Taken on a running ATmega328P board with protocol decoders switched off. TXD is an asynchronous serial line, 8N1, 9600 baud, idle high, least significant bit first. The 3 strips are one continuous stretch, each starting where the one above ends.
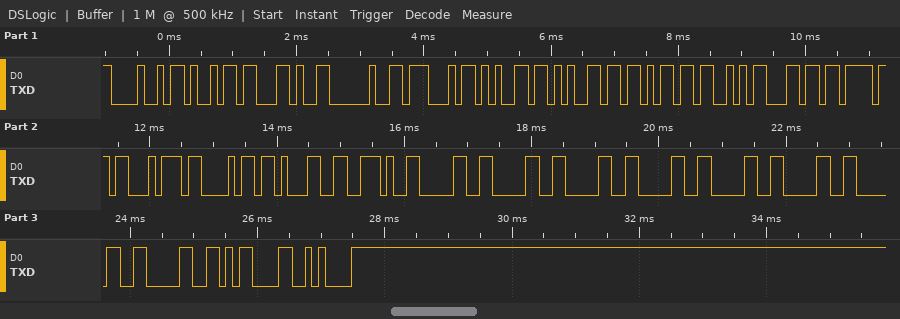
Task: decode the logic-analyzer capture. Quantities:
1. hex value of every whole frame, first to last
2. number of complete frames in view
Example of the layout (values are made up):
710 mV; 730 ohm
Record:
48 69 2C 20 47 65 65 6B 53 6C 6F 74 68 31 2E 30 30 30 30 30 30 30 30 0D 0A; 25
